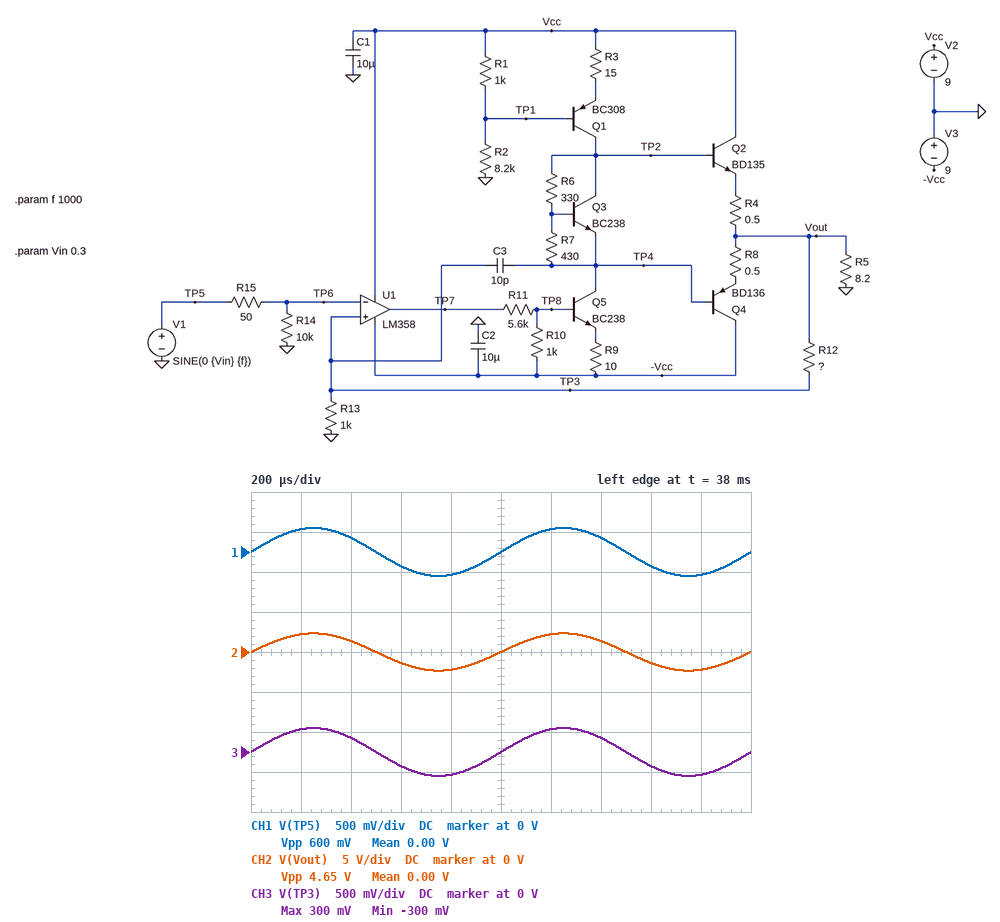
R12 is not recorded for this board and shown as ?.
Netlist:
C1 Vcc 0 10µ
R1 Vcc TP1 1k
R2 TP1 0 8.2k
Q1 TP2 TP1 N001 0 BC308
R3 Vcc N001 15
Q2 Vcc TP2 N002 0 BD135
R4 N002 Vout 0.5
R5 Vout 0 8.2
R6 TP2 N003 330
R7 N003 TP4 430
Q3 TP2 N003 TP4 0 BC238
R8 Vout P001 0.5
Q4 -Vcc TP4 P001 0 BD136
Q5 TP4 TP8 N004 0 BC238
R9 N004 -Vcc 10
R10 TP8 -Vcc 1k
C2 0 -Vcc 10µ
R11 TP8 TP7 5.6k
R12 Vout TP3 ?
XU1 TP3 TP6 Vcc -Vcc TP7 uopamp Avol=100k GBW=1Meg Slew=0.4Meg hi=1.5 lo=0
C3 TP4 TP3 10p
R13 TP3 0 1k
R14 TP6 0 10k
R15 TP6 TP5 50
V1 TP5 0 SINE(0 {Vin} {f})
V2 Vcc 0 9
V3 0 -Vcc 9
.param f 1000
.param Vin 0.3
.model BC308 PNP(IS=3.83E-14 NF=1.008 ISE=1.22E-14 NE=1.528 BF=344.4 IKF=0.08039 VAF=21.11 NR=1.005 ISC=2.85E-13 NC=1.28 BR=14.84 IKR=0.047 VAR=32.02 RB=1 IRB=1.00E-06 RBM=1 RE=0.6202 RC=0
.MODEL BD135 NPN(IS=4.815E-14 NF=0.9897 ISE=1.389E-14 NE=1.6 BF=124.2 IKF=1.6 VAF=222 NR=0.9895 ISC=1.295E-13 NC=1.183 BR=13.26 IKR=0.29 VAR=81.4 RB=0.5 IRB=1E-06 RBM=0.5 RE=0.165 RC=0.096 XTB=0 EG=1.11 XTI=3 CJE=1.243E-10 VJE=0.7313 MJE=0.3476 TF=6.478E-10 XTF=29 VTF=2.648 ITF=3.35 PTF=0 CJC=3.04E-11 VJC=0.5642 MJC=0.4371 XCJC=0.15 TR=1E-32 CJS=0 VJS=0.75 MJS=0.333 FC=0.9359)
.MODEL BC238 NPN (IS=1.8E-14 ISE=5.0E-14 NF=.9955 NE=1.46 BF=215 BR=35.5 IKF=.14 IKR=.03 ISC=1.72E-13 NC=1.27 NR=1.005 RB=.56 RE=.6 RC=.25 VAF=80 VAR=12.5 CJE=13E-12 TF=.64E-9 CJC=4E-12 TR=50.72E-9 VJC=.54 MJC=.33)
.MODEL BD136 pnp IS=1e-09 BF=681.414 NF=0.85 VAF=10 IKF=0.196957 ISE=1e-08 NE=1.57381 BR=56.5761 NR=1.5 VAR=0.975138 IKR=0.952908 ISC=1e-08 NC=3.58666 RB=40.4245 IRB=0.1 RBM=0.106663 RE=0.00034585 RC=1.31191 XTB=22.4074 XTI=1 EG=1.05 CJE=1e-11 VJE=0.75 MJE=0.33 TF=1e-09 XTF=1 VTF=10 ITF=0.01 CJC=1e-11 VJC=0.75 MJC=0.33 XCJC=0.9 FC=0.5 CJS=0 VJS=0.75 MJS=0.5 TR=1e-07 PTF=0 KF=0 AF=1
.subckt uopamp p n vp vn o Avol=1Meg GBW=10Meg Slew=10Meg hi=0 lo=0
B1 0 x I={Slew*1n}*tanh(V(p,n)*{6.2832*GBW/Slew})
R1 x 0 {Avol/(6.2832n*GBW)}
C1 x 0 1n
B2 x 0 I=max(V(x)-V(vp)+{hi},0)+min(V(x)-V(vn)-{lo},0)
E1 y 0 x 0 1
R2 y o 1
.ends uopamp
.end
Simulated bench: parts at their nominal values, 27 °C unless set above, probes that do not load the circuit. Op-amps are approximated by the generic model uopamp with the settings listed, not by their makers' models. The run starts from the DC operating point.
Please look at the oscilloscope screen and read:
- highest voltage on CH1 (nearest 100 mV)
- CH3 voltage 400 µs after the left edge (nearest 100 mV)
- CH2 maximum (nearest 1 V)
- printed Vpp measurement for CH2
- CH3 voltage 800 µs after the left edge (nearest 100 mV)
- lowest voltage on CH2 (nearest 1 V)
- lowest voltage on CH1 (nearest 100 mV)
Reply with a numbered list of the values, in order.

1. 300 mV
2. 200 mV
3. 2 V
4. 4.65 V
5. -300 mV
6. -2 V
7. -300 mV
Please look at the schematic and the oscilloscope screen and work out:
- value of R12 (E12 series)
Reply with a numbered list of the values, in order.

1. 6.8 kΩ
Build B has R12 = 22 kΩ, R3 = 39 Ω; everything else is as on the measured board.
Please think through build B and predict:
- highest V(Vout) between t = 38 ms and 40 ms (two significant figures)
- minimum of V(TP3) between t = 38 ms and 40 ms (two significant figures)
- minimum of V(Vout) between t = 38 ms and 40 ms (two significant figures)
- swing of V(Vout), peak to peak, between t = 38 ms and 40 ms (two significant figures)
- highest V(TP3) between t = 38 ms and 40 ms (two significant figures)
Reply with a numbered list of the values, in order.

1. 5.2 V
2. -300 mV
3. -6.8 V
4. 12 V
5. 230 mV
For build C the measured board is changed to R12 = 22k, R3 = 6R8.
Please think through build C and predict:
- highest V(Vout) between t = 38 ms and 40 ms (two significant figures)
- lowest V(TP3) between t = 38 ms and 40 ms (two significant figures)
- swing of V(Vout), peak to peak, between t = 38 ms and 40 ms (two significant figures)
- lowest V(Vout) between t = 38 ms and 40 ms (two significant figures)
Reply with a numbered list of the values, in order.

1. 6.9 V
2. -290 mV
3. 14 V
4. -6.7 V
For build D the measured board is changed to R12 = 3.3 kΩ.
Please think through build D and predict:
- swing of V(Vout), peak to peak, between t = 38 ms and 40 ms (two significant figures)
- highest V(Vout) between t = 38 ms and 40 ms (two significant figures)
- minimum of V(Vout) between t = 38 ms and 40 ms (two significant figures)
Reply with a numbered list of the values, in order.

1. 2.6 V
2. 1.3 V
3. -1.3 V
